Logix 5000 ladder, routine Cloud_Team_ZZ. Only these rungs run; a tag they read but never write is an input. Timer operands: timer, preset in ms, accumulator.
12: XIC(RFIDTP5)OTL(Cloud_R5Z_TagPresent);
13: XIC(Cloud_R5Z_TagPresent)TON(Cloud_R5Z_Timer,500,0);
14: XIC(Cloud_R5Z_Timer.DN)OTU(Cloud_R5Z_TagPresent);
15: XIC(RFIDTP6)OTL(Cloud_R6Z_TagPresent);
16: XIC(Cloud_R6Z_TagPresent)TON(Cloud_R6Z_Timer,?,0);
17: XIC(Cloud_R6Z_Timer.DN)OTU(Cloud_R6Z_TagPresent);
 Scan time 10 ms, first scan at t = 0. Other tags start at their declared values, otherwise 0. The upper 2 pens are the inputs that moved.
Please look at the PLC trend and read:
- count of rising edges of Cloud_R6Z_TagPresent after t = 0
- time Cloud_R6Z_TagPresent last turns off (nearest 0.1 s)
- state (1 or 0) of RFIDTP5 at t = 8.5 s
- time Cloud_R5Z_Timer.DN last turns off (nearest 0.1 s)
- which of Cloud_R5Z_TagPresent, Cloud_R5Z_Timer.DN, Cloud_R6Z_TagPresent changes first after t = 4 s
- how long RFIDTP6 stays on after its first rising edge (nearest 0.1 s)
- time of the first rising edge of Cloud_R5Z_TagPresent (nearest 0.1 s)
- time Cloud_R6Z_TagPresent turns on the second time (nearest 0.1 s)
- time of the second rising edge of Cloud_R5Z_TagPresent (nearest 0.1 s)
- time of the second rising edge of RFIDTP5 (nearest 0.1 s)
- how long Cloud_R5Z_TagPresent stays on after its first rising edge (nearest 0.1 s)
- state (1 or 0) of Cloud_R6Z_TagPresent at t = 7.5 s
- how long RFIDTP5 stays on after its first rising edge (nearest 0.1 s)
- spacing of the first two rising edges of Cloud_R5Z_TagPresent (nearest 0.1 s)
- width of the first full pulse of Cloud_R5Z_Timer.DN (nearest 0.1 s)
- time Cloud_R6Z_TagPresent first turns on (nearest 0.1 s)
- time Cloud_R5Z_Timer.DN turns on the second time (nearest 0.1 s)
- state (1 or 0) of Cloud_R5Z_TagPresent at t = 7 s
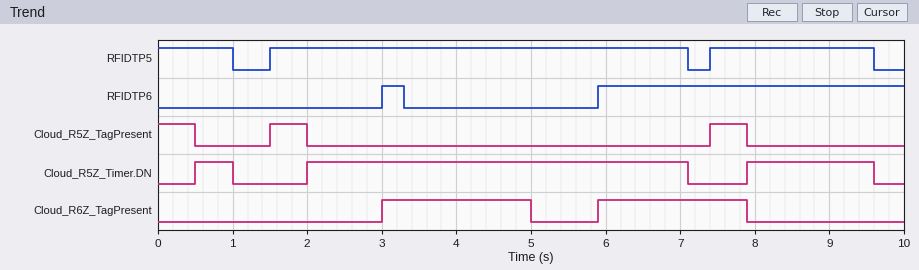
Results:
2
7.9 s
1
9.6 s
Cloud_R6Z_TagPresent
0.3 s
1.5 s
5.9 s
7.4 s
7.4 s
0.5 s
1
5.6 s
5.9 s
0.5 s
3.0 s
2.0 s
0
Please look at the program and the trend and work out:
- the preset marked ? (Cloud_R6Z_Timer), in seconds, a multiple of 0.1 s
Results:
2.0 s
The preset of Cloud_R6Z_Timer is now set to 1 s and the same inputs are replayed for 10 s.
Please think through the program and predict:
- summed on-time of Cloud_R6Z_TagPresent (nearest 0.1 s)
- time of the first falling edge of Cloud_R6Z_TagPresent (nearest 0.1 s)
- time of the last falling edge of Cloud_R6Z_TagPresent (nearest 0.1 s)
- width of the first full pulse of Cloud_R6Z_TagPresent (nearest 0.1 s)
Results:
2.0 s
4.0 s
6.9 s
1.0 s
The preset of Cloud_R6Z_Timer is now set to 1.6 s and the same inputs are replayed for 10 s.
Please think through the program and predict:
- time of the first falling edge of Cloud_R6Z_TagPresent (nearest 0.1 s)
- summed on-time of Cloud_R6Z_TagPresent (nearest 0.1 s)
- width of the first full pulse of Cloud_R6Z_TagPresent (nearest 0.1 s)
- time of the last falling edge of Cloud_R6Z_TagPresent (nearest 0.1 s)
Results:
4.6 s
3.2 s
1.6 s
7.5 s
